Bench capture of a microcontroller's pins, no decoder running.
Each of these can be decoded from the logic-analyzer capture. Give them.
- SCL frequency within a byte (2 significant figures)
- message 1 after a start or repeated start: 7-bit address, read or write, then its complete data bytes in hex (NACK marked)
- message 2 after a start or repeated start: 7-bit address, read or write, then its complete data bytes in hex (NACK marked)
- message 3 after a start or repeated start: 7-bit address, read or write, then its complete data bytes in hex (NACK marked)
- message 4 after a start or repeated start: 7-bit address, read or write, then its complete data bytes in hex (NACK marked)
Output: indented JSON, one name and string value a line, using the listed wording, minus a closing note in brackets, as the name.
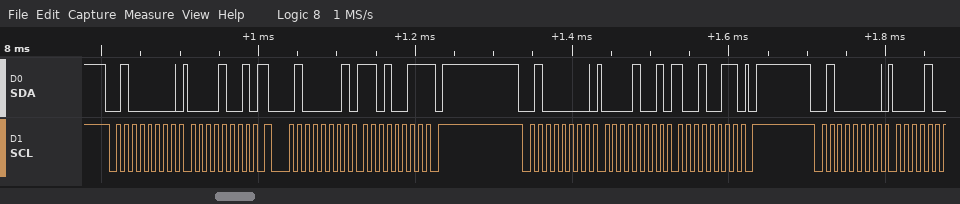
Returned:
{
  "SCL frequency within a byte": "100 kHz",
  "message 1 after a start or repeated start: 7-bit address, read or write, then its complete data bytes in hex": "0x20 write: 09",
  "message 2 after a start or repeated start: 7-bit address, read or write, then its complete data bytes in hex": "0x20 read: D3 NACK",
  "message 3 after a start or repeated start: 7-bit address, read or write, then its complete data bytes in hex": "0x20 write: 09 93",
  "message 4 after a start or repeated start: 7-bit address, read or write, then its complete data bytes in hex": "0x20 write"
}
